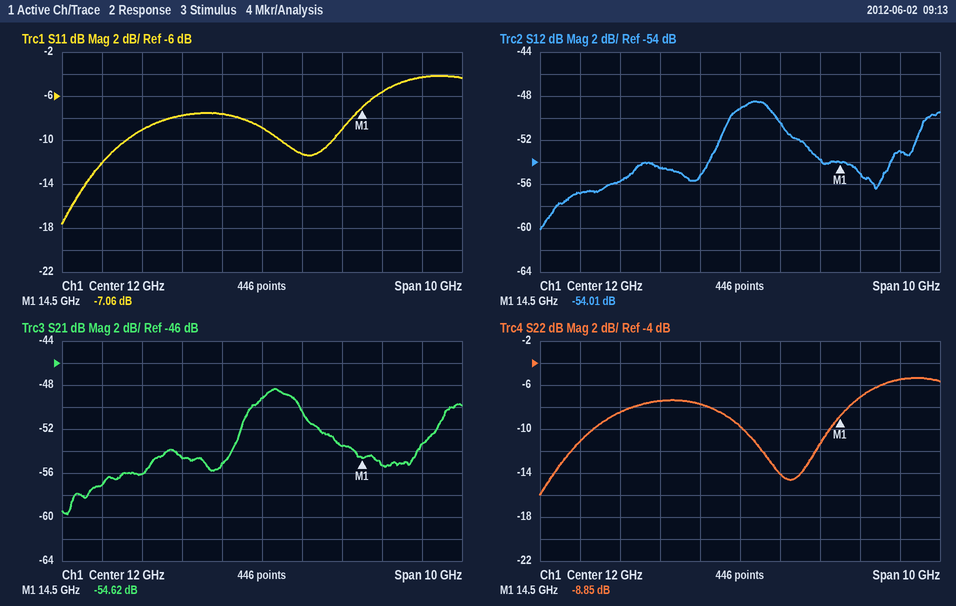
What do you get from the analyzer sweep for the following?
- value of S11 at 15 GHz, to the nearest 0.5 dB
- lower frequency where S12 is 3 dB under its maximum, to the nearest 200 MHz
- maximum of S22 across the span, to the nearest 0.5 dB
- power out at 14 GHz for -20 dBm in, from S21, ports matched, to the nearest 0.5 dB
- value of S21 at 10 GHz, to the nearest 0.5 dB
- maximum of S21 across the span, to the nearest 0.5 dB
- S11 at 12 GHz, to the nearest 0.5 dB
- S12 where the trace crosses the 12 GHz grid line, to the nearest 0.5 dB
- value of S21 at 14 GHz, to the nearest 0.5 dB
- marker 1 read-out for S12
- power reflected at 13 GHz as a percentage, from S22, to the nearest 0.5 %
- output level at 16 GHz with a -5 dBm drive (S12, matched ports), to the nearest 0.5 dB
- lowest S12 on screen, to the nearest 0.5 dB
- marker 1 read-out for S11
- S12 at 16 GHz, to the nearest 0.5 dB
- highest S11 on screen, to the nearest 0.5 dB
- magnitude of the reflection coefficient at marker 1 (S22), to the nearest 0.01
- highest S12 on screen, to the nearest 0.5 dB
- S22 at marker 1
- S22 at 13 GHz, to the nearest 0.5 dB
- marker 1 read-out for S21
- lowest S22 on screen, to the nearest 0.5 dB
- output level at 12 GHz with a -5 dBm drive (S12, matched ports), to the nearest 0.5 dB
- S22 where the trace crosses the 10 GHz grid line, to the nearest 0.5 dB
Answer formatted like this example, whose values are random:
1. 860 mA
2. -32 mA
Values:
1. -5.5 dB
2. 11.6 GHz
3. -5.5 dB
4. -73.5 dBm
5. -54.5 dB
6. -48.5 dB
7. -9.0 dB
8. -49.0 dB
9. -53.5 dB
10. -54.01 dB
11. 4.0 %
12. -58.0 dBm
13. -60.0 dB
14. -7.06 dB
15. -53.0 dB
16. -4.0 dB
17. 0.36
18. -48.5 dB
19. -8.85 dB
20. -14.0 dB
21. -54.62 dB
22. -16.0 dB
23. -54.0 dBm
24. -7.5 dB
